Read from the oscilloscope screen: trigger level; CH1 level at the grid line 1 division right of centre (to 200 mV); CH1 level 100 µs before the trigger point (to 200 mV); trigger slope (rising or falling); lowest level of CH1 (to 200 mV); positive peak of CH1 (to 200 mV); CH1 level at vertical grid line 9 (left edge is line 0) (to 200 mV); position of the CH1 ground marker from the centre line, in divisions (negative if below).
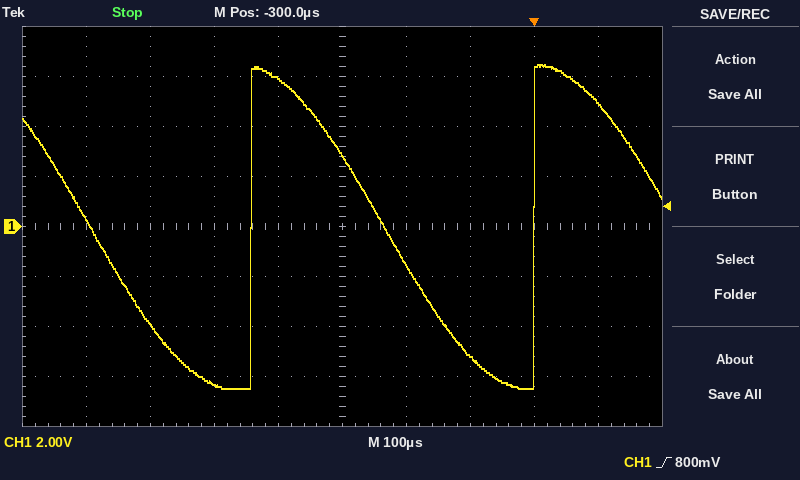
800 mV
-1.6 V
-5.2 V
rising
-6.4 V
6.4 V
5.0 V
0.0 div
